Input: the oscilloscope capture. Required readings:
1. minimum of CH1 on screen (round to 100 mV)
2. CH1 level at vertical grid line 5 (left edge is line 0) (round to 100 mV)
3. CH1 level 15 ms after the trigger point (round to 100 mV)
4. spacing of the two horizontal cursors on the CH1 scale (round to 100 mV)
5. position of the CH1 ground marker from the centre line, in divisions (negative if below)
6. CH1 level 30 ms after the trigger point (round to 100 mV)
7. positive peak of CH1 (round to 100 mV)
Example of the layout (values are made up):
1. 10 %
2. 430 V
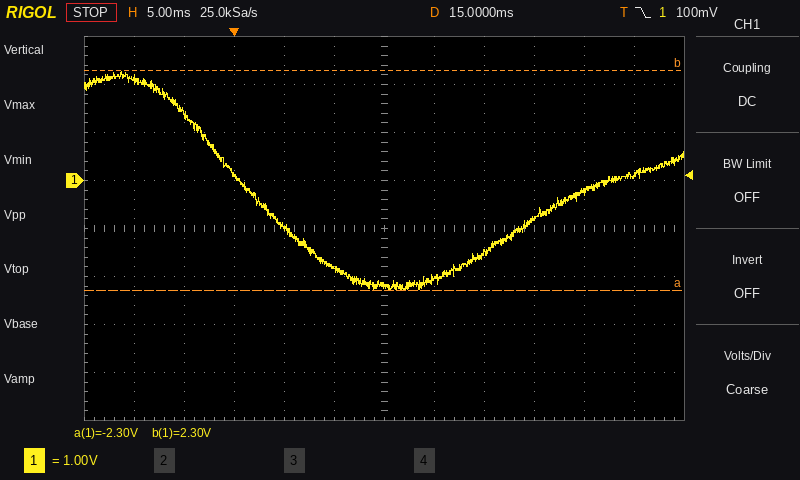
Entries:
1. -2.3 V
2. -1.8 V
3. -2.2 V
4. 4.6 V
5. +1.0 div
6. -800 mV
7. 2.3 V
